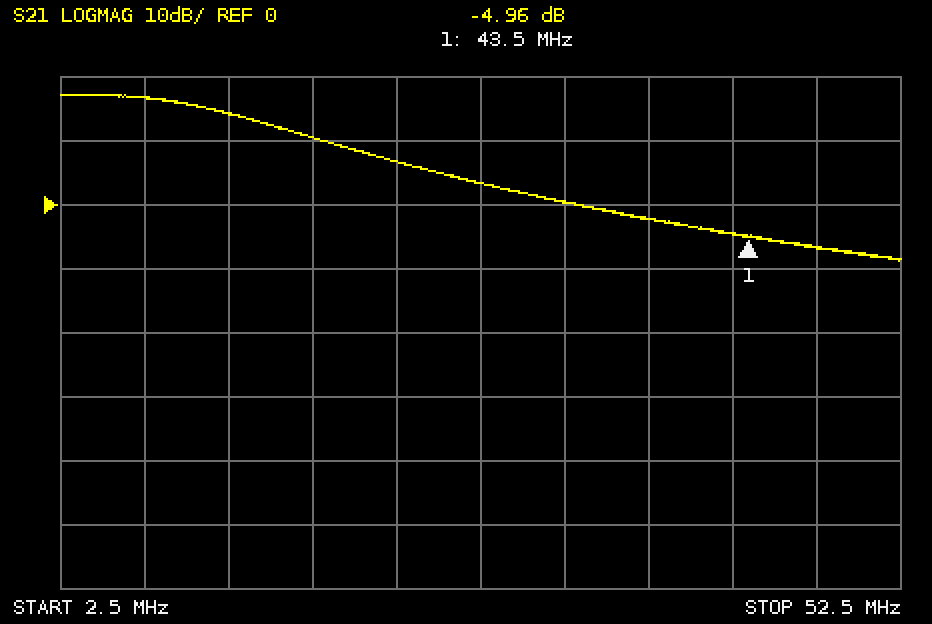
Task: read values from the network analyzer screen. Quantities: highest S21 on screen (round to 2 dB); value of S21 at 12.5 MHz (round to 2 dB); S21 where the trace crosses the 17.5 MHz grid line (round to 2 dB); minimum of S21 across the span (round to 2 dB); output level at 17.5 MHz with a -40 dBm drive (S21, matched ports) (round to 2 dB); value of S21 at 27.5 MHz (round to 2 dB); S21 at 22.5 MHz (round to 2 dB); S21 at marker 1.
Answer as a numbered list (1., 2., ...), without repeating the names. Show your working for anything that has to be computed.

1. 18 dB
2. 14 dB
3. 10 dB
4. -8 dB
5. -40 dBm + (10 dB) = -30 dBm
6. 4 dB
7. 6 dB
8. -4.96 dB
